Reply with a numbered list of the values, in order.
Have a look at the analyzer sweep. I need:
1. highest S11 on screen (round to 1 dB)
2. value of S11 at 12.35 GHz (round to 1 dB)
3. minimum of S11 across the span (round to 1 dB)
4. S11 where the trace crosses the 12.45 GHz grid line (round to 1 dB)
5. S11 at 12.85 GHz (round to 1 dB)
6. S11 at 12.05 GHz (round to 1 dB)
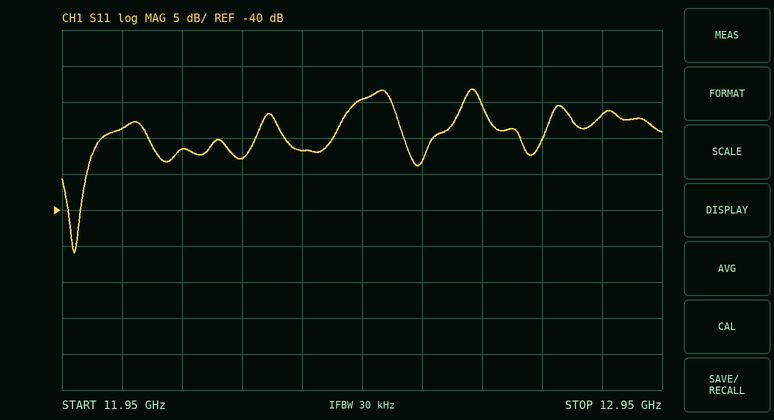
1. -23 dB
2. -32 dB
3. -46 dB
4. -25 dB
5. -27 dB
6. -29 dB
